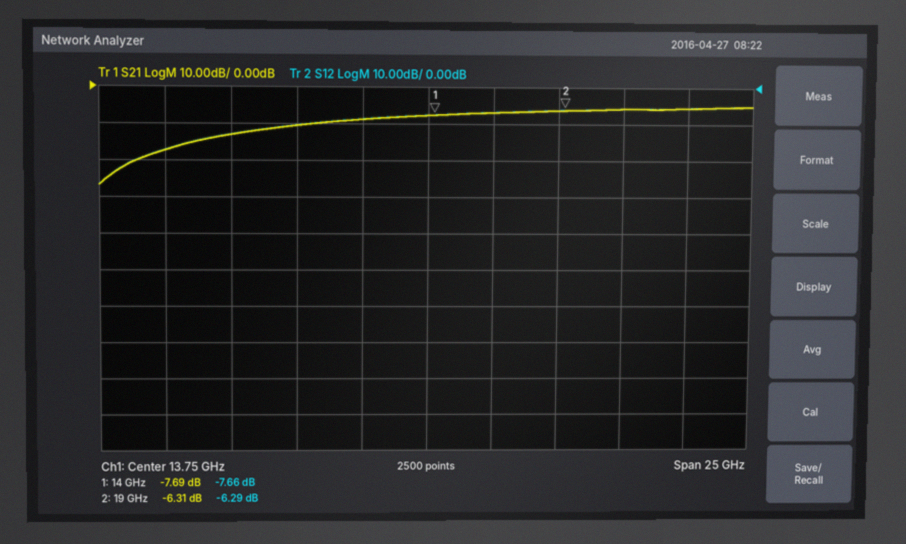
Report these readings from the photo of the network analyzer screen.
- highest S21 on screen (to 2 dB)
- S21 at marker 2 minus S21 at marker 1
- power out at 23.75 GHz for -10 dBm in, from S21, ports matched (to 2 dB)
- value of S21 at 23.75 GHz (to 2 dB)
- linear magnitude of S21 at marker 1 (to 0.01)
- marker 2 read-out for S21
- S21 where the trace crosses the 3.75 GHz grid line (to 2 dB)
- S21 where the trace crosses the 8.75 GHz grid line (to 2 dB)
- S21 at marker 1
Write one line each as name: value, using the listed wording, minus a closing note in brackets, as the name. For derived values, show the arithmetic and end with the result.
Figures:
highest S21 on screen: -6 dB
S21 at marker 2 minus S21 at marker 1: -6.31 − (-7.69) = 1.38 dB
power out at 23.75 GHz for -10 dBm in, from S21, ports matched: -10 dBm + (-6 dB) = -16 dBm
value of S21 at 23.75 GHz: -6 dB
linear magnitude of S21 at marker 1: 10^(-7.69/20) ≈ 0.41
marker 2 read-out for S21: -6.31 dB
S21 where the trace crosses the 3.75 GHz grid line: -18 dB
S21 where the trace crosses the 8.75 GHz grid line: -10 dB
S21 at marker 1: -7.69 dB
